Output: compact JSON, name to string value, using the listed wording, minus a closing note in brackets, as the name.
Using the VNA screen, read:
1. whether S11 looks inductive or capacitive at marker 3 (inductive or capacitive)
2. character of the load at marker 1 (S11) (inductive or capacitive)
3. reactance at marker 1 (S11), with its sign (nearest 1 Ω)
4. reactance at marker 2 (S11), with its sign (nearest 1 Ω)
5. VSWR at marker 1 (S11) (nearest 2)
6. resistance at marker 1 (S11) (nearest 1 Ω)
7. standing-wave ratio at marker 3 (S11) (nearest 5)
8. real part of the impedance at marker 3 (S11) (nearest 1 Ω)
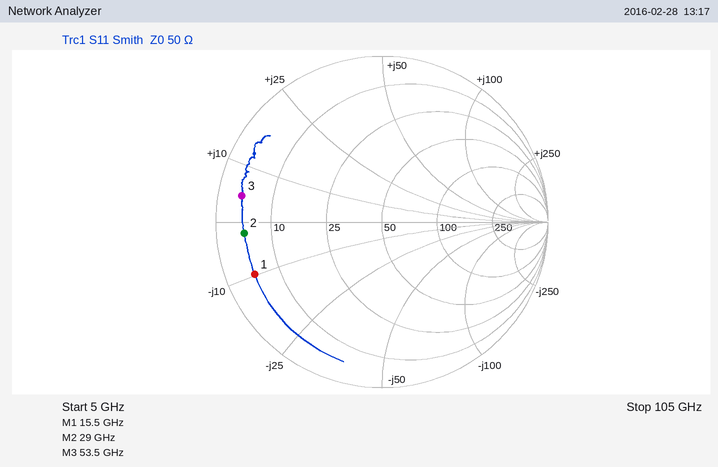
{"whether S11 looks inductive or capacitive at marker 3": "inductive", "character of the load at marker 1 (S11)": "capacitive", "reactance at marker 1 (S11), with its sign": "-10 Ω", "reactance at marker 2 (S11), with its sign": "-2 Ω", "VSWR at marker 1 (S11)": "10", "resistance at marker 1 (S11)": "5 Ω", "standing-wave ratio at marker 3 (S11)": "15", "real part of the impedance at marker 3 (S11)": "4 Ω"}
